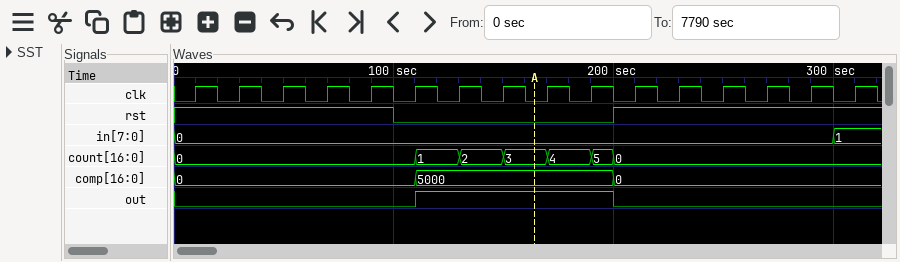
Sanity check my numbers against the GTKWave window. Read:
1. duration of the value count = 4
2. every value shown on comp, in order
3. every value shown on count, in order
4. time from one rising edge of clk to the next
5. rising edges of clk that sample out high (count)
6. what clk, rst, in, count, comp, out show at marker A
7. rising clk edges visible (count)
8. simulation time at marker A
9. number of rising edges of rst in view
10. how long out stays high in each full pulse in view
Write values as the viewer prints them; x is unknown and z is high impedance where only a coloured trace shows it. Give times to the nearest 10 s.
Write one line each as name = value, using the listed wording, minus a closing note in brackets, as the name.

duration of the value count = 4 = 20 s
every value shown on comp, in order = 0, 5000, 0
every value shown on count, in order = 0, 1, 2, 3, 4, 5, 0
time from one rising edge of clk to the next = 20 s
rising edges of clk that sample out high = 4
what clk, rst, in, count, comp, out show at marker A = clk=0, rst=0, in=0, count=3, comp=5000, out=1
rising clk edges visible = 16
simulation time at marker A = 160 s
number of rising edges of rst in view = 1
how long out stays high in each full pulse in view = 90 s
